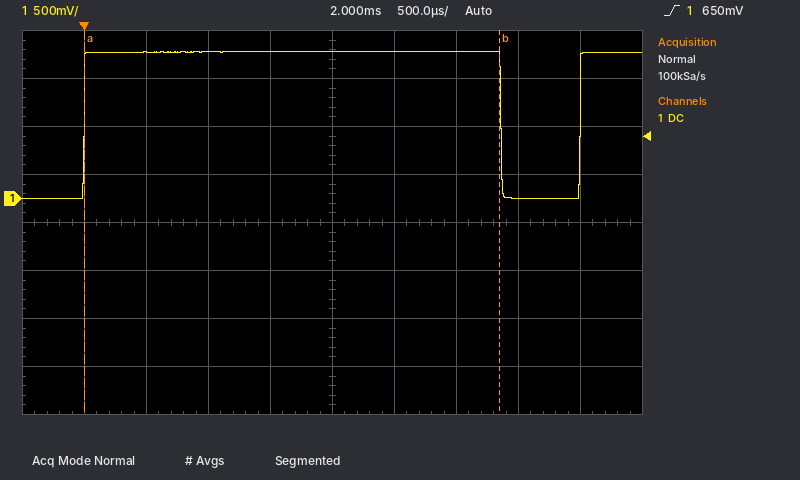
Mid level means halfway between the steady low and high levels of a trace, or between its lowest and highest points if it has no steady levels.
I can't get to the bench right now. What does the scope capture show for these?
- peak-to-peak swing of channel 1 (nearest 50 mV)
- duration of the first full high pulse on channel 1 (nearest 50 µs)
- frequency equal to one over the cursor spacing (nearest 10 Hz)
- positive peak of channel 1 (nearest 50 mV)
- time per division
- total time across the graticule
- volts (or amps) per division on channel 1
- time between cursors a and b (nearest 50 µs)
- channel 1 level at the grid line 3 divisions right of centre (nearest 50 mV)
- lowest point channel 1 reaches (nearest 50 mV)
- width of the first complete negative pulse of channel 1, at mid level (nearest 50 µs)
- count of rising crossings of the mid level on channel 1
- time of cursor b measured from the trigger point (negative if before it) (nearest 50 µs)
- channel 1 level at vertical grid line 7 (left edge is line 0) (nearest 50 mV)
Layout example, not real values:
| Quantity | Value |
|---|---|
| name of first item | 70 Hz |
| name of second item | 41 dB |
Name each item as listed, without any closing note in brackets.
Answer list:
| Quantity | Value |
|---|---|
| peak-to-peak swing of channel 1 | 1.55 V |
| duration of the first full high pulse on channel 1 | 3.35 ms |
| frequency equal to one over the cursor spacing | 300 Hz |
| positive peak of channel 1 | 1.55 V |
| time per division | 500 µs |
| total time across the graticule | 5 ms |
| volts (or amps) per division on channel 1 | 500 mV |
| time between cursors a and b | 3.35 ms |
| channel 1 level at the grid line 3 divisions right of centre | 0 mV |
| lowest point channel 1 reaches | 0 mV |
| width of the first complete negative pulse of channel 1, at mid level | 650 µs |
| count of rising crossings of the mid level on channel 1 | 2 |
| time of cursor b measured from the trigger point (negative if before it) | +3.35 ms |
| channel 1 level at vertical grid line 7 (left edge is line 0) | 1.55 V |
